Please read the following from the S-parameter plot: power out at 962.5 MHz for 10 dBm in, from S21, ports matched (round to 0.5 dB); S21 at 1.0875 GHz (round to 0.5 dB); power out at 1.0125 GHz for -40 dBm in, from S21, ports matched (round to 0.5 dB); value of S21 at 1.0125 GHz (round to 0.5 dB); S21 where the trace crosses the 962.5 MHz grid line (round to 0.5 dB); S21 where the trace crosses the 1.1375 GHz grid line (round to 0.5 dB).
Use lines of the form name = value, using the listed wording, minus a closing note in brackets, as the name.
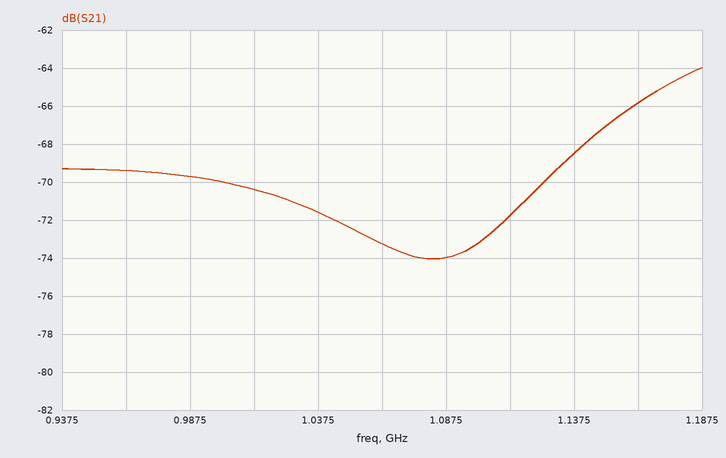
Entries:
power out at 962.5 MHz for 10 dBm in, from S21, ports matched = -59.5 dBm
S21 at 1.0875 GHz = -74.0 dB
power out at 1.0125 GHz for -40 dBm in, from S21, ports matched = -110.5 dBm
value of S21 at 1.0125 GHz = -70.5 dB
S21 where the trace crosses the 962.5 MHz grid line = -69.5 dB
S21 where the trace crosses the 1.1375 GHz grid line = -68.5 dB
